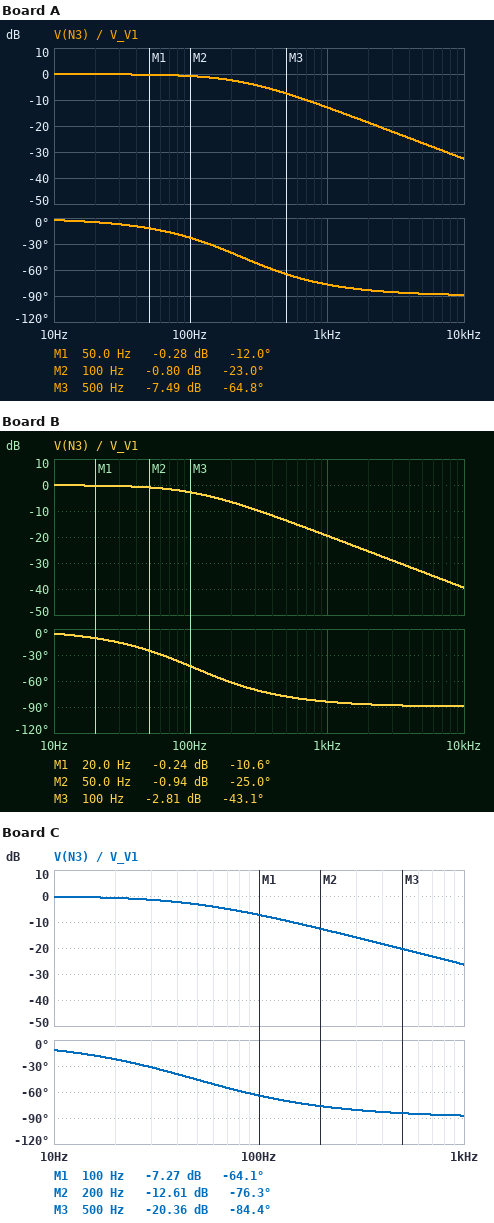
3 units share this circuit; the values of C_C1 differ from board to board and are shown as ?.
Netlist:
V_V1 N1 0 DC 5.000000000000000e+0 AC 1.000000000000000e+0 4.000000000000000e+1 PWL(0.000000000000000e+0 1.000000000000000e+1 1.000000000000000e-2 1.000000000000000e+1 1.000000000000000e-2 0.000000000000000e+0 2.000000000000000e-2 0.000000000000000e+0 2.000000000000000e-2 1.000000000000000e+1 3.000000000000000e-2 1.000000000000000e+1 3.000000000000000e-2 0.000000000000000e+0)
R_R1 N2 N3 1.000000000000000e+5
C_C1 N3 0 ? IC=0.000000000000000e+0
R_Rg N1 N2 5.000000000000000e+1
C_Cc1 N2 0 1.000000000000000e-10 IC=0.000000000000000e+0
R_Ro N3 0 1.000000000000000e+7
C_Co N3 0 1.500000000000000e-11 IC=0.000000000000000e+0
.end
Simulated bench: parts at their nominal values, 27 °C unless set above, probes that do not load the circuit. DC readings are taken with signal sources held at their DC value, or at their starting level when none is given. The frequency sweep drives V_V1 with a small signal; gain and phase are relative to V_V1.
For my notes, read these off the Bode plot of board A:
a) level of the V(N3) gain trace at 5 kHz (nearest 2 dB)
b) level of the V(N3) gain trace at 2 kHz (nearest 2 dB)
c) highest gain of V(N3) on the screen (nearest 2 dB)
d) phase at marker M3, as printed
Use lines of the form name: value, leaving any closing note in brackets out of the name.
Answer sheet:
level of the V(N3) gain trace at 5 kHz: -26 dB
level of the V(N3) gain trace at 2 kHz: -18 dB
highest gain of V(N3) on the screen: 0 dB
phase at marker M3, as printed: -64.8 deg
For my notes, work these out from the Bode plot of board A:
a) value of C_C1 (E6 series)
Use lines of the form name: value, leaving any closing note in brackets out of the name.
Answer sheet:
value of C_C1: 6.8 nF
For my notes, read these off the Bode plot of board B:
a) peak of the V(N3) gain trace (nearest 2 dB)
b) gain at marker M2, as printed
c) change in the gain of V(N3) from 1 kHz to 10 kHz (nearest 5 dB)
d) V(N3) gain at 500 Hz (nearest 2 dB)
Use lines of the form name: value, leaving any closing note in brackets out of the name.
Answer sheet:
peak of the V(N3) gain trace: 0 dB
gain at marker M2, as printed: -0.94 dB
change in the gain of V(N3) from 1 kHz to 10 kHz: -20 dB
V(N3) gain at 500 Hz: -14 dB
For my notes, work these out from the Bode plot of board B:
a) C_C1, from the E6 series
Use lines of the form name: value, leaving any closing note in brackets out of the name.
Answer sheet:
C_C1, from the E6 series: 15 nF
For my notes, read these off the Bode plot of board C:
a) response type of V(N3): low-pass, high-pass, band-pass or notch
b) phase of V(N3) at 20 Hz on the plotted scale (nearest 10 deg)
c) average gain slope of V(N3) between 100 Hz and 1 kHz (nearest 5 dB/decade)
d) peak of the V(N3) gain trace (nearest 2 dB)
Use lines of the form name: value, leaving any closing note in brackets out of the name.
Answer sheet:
response type of V(N3): low-pass, high-pass, band-pass or notch: low-pass
phase of V(N3) at 20 Hz on the plotted scale: -20 deg
average gain slope of V(N3) between 100 Hz and 1 kHz: -20 dB/decade
peak of the V(N3) gain trace: 0 dB
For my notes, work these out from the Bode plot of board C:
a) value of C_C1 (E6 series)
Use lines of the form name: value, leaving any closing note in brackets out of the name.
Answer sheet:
value of C_C1: 33 nF
